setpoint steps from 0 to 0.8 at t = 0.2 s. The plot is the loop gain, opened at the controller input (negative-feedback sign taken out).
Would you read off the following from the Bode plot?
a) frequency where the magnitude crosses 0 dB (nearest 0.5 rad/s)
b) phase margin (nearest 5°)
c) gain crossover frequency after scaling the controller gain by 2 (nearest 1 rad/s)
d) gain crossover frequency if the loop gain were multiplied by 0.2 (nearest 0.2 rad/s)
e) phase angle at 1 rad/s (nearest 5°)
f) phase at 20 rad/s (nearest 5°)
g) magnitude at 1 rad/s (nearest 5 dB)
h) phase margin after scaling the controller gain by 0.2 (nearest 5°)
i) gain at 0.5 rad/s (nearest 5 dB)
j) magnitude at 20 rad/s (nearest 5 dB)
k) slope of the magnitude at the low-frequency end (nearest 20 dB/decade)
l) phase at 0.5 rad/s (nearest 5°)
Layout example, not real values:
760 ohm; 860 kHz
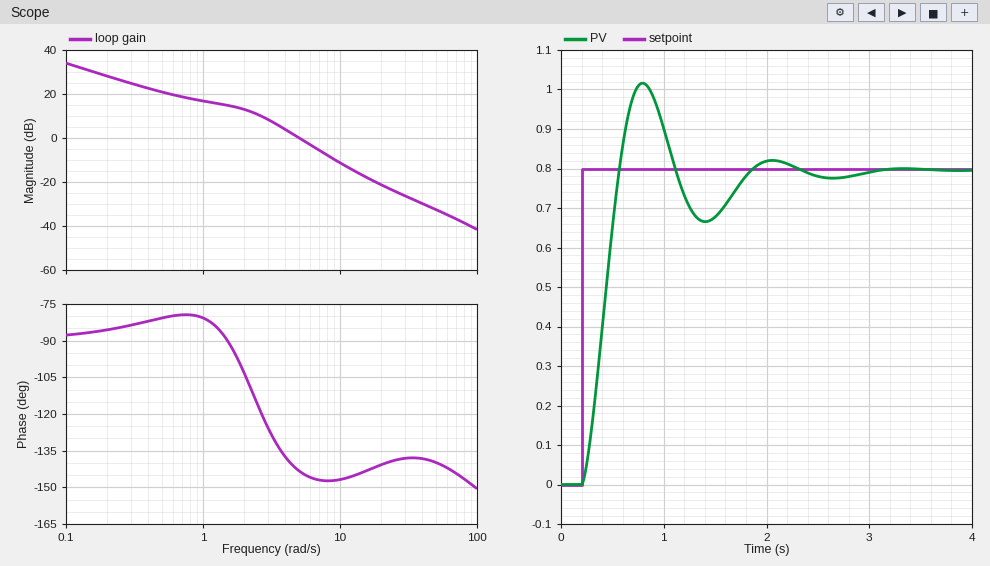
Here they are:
5.0 rad/s; 35°; 7 rad/s; 1.8 rad/s; -80°; -140°; 15 dB; 85°; 20 dB; -20 dB; -20 dB/decade; -80°
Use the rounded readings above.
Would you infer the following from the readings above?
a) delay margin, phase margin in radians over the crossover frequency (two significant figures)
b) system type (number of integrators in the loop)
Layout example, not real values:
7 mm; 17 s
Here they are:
0.12 s; 1
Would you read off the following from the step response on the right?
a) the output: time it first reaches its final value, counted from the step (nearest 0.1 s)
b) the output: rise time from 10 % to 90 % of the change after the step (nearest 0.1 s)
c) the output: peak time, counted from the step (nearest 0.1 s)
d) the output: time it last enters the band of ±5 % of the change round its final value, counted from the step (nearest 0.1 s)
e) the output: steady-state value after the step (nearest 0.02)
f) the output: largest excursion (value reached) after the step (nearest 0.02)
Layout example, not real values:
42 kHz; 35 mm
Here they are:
0.4 s; 0.3 s; 0.6 s; 1.5 s; 0.80; 1.02
